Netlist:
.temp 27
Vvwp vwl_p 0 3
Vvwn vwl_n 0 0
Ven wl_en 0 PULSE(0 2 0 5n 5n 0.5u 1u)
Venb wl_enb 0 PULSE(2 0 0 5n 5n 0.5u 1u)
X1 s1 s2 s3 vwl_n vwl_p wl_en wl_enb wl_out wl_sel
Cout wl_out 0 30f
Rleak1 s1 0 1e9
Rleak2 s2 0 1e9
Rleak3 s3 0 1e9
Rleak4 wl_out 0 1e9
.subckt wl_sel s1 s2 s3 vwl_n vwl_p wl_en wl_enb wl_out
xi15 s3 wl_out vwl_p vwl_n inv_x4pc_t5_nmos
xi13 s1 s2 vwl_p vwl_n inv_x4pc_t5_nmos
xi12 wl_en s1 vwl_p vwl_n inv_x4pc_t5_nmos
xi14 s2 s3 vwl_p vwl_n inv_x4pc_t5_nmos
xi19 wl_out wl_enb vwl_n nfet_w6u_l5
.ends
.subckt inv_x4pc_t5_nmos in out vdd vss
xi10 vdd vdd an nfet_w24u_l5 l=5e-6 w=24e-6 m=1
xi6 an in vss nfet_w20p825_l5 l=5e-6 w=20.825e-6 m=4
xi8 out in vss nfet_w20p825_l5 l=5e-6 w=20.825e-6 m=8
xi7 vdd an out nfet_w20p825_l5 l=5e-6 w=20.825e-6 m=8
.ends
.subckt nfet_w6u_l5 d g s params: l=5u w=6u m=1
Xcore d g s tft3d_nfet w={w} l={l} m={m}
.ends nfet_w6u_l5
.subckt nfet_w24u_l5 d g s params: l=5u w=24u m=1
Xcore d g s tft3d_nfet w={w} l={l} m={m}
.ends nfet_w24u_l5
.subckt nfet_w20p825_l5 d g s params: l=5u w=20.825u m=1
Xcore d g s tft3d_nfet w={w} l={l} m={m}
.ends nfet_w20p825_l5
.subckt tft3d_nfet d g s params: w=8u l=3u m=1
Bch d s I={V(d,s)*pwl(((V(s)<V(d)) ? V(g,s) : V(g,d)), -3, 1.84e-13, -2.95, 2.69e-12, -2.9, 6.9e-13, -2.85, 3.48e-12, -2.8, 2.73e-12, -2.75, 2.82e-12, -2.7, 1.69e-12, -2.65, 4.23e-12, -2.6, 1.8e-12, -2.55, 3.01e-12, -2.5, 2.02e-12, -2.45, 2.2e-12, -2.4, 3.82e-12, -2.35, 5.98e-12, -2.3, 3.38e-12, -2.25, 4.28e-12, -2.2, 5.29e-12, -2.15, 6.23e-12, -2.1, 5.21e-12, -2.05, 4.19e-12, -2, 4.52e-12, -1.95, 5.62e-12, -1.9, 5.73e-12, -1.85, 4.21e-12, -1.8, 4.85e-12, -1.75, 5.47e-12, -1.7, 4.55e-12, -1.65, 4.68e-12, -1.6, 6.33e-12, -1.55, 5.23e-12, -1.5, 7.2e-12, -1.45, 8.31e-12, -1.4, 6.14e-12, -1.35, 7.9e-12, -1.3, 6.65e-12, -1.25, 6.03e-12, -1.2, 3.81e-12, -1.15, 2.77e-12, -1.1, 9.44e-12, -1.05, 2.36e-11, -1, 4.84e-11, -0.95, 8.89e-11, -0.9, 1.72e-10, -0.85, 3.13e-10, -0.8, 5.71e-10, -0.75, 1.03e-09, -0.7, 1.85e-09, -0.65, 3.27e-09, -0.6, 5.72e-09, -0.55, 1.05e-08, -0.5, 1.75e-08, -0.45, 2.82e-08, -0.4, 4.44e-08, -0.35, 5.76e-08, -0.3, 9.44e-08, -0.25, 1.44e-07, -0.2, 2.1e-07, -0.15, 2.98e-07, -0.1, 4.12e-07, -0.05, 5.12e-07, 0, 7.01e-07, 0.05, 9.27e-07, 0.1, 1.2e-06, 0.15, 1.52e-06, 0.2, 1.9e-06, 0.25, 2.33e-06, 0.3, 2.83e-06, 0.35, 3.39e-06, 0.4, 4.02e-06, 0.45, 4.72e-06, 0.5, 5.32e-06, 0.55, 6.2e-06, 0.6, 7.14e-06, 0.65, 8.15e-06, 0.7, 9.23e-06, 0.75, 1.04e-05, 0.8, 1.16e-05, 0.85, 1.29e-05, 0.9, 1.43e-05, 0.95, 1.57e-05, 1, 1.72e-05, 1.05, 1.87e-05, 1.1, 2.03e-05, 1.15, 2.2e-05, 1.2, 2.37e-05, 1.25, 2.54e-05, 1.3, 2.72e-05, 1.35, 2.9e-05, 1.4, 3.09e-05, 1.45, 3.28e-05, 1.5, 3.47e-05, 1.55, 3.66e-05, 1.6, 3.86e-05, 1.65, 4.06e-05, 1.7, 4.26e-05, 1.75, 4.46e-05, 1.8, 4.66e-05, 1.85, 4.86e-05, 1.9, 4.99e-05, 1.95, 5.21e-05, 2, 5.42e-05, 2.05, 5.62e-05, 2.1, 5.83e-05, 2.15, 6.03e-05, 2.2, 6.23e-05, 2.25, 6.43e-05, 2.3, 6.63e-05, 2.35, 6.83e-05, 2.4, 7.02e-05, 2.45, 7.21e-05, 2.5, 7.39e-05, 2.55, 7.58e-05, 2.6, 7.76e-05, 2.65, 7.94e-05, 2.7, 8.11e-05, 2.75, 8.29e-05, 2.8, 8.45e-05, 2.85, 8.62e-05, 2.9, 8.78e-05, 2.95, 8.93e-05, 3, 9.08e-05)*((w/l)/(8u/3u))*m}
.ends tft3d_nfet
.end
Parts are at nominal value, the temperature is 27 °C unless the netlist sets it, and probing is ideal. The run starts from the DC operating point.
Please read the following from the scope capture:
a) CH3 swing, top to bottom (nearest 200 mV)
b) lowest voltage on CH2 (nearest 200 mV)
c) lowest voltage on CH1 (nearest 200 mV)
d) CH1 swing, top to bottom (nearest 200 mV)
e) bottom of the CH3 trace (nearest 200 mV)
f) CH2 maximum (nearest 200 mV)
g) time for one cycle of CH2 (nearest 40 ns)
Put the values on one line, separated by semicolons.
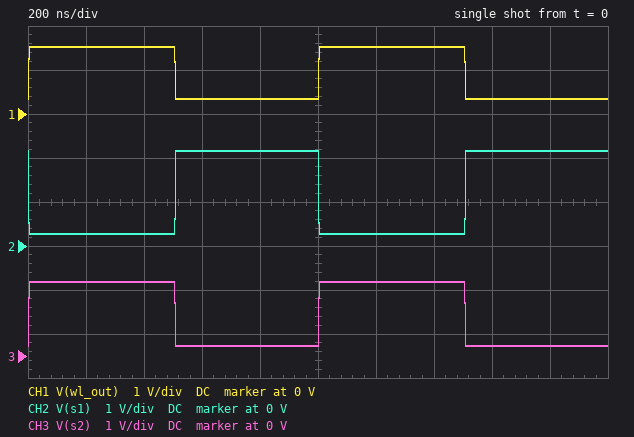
1.4 V; 200 mV; 400 mV; 1.2 V; 200 mV; 2.2 V; 1.00 µs
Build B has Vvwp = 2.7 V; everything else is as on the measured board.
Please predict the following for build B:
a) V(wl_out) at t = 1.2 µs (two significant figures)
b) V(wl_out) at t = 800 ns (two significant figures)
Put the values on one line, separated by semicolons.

1.4 V; 320 mV
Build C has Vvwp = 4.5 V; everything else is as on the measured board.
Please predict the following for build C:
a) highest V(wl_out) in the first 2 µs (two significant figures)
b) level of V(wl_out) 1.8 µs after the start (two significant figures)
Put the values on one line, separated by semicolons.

2.0 V; 460 mV
